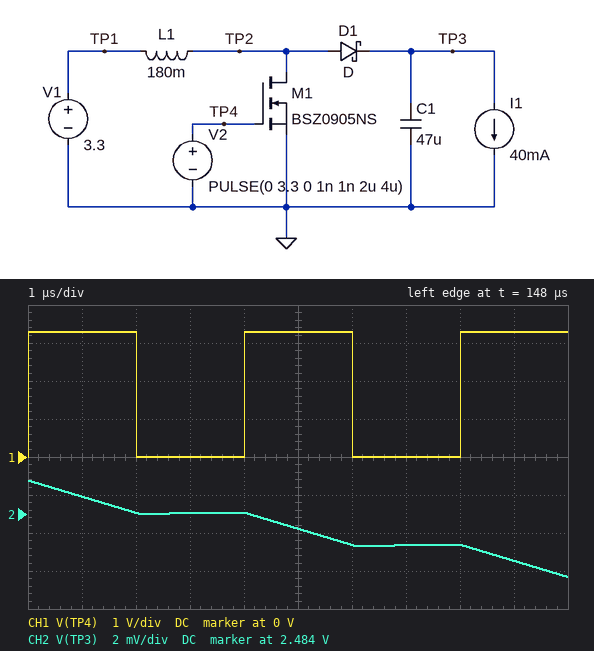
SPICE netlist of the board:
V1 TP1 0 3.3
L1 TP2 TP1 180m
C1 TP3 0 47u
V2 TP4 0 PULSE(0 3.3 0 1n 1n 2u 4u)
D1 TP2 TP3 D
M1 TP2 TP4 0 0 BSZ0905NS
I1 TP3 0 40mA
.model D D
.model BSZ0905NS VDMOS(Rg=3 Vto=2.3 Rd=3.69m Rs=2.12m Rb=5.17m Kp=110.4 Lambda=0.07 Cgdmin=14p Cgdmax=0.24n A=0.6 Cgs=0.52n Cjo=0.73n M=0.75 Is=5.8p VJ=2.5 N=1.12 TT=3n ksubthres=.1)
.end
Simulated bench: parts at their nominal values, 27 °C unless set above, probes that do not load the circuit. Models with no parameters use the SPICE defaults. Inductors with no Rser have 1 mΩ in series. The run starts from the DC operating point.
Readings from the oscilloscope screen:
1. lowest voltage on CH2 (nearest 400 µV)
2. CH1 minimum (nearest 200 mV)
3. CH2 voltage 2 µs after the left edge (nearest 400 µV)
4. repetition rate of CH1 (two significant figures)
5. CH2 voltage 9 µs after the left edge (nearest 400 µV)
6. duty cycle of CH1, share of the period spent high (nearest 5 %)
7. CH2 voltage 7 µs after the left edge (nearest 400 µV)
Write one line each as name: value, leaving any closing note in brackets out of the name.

lowest voltage on CH2: 2.4808 V
CH1 minimum: 0 V
CH2 voltage 2 µs after the left edge: 2.4840 V
repetition rate of CH1: 250 kHz
CH2 voltage 9 µs after the left edge: 2.4816 V
duty cycle of CH1, share of the period spent high: 50 %
CH2 voltage 7 µs after the left edge: 2.4824 V
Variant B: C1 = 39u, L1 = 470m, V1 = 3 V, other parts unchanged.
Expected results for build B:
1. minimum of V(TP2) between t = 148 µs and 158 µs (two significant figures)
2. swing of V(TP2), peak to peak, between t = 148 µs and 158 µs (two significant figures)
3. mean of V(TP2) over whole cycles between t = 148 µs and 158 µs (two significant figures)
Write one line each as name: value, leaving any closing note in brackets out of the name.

minimum of V(TP2) between t = 148 µs and 158 µs: -260 mV
swing of V(TP2), peak to peak, between t = 148 µs and 158 µs: 3.2 V
mean of V(TP2) over whole cycles between t = 148 µs and 158 µs: 1.4 V
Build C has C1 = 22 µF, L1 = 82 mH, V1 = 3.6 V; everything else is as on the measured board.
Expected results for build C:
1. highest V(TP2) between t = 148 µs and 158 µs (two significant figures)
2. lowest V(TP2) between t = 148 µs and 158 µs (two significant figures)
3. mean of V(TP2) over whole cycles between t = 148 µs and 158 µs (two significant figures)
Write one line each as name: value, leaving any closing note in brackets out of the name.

highest V(TP2) between t = 148 µs and 158 µs: 3.5 V
lowest V(TP2) between t = 148 µs and 158 µs: -250 mV
mean of V(TP2) over whole cycles between t = 148 µs and 158 µs: 1.7 V
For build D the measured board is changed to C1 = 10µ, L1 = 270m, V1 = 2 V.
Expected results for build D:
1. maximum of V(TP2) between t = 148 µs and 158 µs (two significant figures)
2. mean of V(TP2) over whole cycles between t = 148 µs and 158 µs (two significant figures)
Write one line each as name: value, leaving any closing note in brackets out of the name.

maximum of V(TP2) between t = 148 µs and 158 µs: 1.7 V
mean of V(TP2) over whole cycles between t = 148 µs and 158 µs: 830 mV
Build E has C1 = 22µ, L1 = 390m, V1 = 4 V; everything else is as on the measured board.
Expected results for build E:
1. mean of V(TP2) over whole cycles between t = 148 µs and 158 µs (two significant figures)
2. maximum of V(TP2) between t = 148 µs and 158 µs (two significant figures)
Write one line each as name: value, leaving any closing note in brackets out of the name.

mean of V(TP2) over whole cycles between t = 148 µs and 158 µs: 1.9 V
maximum of V(TP2) between t = 148 µs and 158 µs: 3.9 V
